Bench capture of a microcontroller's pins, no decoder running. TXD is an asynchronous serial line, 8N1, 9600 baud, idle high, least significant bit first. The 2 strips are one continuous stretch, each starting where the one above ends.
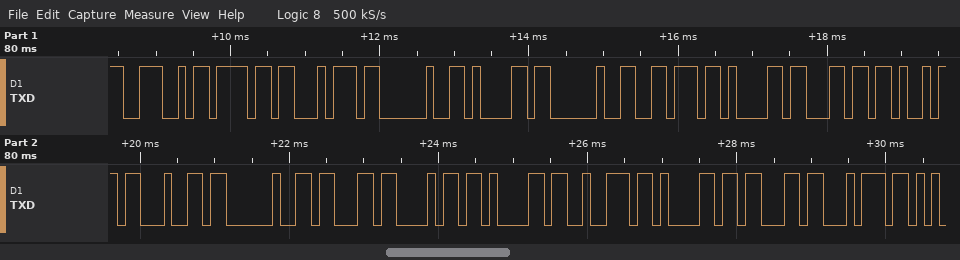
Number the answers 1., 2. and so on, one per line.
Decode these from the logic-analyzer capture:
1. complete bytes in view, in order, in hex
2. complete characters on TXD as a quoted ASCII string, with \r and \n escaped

1. 0x4E 0x6F 0x74 0x20 0x61 0x20 0x76 0x61 0x6C 0x69 0x64 0x20 0x63 0x68 0x61 0x72 0x61 0x63 0x74
2. "Not a valid charact"
